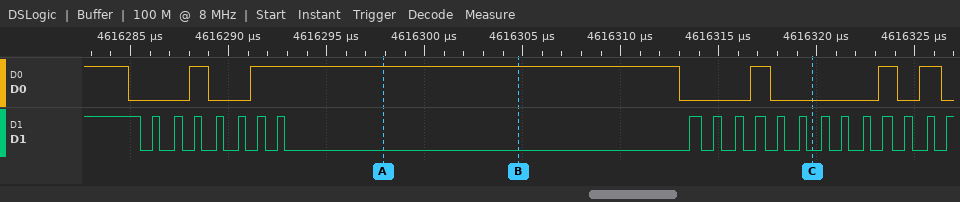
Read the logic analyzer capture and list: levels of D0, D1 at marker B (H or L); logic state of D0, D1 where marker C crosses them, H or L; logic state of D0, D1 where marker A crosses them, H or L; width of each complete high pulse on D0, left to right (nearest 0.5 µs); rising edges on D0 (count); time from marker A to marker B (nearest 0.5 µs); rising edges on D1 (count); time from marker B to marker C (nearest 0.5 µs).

D0=H, D1=L
D0=L, D1=L
D0=H, D1=L
1 µs, 22 µs, 1 µs, 1 µs, 1 µs
5
7 µs
20
15 µs
